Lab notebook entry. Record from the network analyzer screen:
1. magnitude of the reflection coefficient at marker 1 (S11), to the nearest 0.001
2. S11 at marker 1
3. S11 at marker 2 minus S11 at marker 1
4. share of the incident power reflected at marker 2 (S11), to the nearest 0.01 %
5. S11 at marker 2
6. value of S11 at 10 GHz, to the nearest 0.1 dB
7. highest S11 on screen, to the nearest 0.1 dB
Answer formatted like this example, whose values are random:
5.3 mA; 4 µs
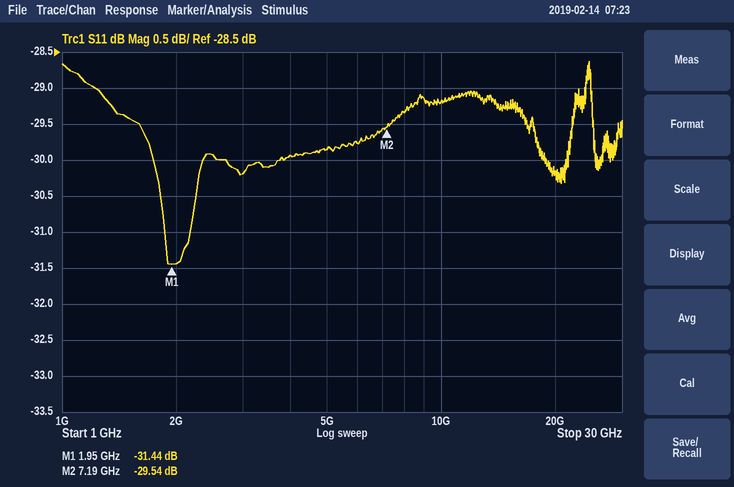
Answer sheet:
0.027; -31.44 dB; 1.90 dB; 0.11 %; -29.54 dB; -29.2 dB; -28.6 dB
